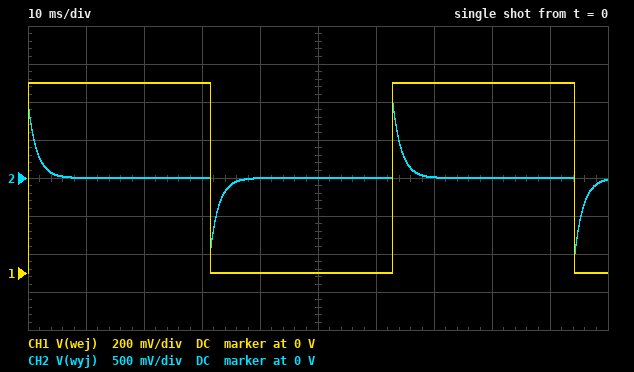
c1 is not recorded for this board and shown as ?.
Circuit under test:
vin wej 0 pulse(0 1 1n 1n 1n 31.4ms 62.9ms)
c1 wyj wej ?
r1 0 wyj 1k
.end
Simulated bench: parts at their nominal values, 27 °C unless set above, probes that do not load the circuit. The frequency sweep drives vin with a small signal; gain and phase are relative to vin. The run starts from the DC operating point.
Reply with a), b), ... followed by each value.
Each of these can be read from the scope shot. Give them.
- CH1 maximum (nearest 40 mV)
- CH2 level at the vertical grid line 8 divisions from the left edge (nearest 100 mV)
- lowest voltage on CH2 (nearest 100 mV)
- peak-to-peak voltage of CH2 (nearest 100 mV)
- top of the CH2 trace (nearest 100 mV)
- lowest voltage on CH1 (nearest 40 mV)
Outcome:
a) 1.00 V
b) 0 V
c) -1.0 V
d) 2.0 V
e) 1.0 V
f) 0 V
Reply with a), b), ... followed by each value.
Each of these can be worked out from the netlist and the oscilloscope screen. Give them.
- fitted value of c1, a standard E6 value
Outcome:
a) 1.5 µF
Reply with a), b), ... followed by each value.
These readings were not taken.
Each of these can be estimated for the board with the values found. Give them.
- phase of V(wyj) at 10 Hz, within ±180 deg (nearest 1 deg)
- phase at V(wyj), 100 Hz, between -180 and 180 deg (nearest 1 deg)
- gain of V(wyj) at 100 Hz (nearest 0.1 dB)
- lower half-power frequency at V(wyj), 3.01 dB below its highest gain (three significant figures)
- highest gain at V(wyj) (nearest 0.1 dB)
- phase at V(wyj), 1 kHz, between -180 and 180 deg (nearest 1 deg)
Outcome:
a) 85 deg
b) 47 deg
c) -3.3 dB
d) 106 Hz
e) 0 dB
f) 6 deg
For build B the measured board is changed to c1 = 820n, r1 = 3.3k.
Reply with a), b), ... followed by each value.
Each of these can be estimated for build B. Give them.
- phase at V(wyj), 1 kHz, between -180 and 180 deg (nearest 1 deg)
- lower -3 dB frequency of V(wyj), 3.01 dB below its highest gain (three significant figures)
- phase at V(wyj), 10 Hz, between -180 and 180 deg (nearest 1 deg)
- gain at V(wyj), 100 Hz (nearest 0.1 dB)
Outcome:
a) 3 deg
b) 58.8 Hz
c) 80 deg
d) -1.3 dB
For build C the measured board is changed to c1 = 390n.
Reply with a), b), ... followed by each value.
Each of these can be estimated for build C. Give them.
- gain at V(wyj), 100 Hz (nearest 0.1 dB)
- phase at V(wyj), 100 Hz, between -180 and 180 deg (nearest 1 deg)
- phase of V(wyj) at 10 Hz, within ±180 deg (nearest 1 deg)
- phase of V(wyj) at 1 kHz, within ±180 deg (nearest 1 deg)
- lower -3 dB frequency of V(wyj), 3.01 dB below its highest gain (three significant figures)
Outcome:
a) -12.5 dB
b) 76 deg
c) 89 deg
d) 22 deg
e) 408 Hz
